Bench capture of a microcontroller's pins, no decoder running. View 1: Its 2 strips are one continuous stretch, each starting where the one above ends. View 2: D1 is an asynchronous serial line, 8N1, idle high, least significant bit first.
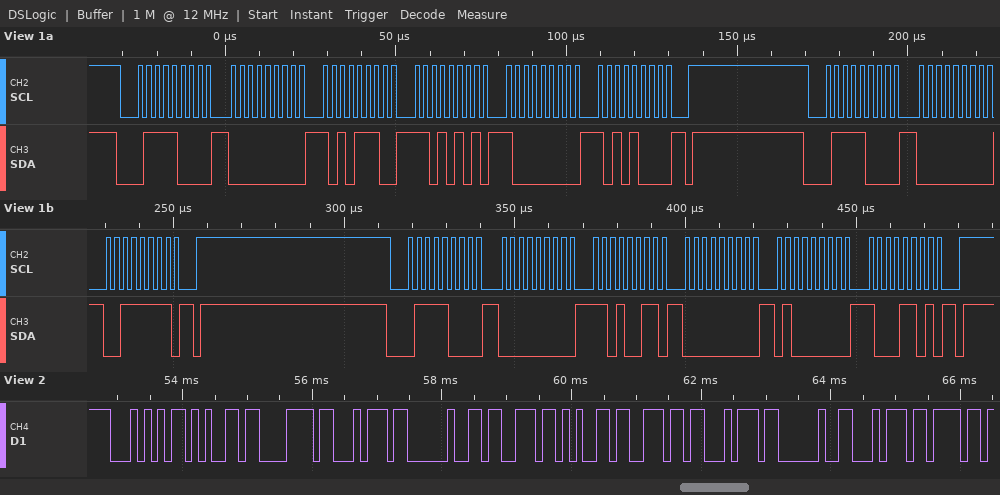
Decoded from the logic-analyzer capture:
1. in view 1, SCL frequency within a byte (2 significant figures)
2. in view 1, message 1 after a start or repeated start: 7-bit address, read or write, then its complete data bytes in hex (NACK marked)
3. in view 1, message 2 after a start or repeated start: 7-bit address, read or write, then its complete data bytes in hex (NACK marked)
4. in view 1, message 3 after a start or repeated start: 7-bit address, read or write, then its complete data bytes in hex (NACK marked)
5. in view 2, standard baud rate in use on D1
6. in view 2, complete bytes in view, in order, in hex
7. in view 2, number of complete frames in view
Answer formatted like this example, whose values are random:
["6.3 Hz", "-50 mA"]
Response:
["400 kHz", "0x3C write: 00 AE D5 80 A8", "0x3C write: 00 3F", "0x3C write: 00 D3 00 40 8D", "9600 baud", "0x54 0x65 0x78 0x74 0x20 0x73 0x65 0x6E 0x74 0x20 0x74 0x6F", "12"]
